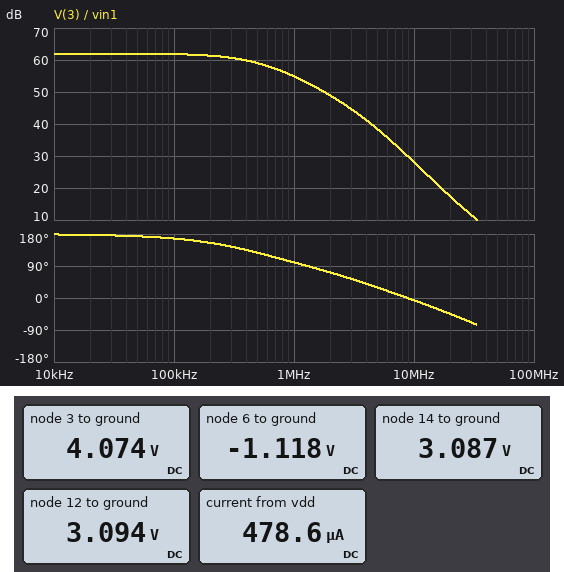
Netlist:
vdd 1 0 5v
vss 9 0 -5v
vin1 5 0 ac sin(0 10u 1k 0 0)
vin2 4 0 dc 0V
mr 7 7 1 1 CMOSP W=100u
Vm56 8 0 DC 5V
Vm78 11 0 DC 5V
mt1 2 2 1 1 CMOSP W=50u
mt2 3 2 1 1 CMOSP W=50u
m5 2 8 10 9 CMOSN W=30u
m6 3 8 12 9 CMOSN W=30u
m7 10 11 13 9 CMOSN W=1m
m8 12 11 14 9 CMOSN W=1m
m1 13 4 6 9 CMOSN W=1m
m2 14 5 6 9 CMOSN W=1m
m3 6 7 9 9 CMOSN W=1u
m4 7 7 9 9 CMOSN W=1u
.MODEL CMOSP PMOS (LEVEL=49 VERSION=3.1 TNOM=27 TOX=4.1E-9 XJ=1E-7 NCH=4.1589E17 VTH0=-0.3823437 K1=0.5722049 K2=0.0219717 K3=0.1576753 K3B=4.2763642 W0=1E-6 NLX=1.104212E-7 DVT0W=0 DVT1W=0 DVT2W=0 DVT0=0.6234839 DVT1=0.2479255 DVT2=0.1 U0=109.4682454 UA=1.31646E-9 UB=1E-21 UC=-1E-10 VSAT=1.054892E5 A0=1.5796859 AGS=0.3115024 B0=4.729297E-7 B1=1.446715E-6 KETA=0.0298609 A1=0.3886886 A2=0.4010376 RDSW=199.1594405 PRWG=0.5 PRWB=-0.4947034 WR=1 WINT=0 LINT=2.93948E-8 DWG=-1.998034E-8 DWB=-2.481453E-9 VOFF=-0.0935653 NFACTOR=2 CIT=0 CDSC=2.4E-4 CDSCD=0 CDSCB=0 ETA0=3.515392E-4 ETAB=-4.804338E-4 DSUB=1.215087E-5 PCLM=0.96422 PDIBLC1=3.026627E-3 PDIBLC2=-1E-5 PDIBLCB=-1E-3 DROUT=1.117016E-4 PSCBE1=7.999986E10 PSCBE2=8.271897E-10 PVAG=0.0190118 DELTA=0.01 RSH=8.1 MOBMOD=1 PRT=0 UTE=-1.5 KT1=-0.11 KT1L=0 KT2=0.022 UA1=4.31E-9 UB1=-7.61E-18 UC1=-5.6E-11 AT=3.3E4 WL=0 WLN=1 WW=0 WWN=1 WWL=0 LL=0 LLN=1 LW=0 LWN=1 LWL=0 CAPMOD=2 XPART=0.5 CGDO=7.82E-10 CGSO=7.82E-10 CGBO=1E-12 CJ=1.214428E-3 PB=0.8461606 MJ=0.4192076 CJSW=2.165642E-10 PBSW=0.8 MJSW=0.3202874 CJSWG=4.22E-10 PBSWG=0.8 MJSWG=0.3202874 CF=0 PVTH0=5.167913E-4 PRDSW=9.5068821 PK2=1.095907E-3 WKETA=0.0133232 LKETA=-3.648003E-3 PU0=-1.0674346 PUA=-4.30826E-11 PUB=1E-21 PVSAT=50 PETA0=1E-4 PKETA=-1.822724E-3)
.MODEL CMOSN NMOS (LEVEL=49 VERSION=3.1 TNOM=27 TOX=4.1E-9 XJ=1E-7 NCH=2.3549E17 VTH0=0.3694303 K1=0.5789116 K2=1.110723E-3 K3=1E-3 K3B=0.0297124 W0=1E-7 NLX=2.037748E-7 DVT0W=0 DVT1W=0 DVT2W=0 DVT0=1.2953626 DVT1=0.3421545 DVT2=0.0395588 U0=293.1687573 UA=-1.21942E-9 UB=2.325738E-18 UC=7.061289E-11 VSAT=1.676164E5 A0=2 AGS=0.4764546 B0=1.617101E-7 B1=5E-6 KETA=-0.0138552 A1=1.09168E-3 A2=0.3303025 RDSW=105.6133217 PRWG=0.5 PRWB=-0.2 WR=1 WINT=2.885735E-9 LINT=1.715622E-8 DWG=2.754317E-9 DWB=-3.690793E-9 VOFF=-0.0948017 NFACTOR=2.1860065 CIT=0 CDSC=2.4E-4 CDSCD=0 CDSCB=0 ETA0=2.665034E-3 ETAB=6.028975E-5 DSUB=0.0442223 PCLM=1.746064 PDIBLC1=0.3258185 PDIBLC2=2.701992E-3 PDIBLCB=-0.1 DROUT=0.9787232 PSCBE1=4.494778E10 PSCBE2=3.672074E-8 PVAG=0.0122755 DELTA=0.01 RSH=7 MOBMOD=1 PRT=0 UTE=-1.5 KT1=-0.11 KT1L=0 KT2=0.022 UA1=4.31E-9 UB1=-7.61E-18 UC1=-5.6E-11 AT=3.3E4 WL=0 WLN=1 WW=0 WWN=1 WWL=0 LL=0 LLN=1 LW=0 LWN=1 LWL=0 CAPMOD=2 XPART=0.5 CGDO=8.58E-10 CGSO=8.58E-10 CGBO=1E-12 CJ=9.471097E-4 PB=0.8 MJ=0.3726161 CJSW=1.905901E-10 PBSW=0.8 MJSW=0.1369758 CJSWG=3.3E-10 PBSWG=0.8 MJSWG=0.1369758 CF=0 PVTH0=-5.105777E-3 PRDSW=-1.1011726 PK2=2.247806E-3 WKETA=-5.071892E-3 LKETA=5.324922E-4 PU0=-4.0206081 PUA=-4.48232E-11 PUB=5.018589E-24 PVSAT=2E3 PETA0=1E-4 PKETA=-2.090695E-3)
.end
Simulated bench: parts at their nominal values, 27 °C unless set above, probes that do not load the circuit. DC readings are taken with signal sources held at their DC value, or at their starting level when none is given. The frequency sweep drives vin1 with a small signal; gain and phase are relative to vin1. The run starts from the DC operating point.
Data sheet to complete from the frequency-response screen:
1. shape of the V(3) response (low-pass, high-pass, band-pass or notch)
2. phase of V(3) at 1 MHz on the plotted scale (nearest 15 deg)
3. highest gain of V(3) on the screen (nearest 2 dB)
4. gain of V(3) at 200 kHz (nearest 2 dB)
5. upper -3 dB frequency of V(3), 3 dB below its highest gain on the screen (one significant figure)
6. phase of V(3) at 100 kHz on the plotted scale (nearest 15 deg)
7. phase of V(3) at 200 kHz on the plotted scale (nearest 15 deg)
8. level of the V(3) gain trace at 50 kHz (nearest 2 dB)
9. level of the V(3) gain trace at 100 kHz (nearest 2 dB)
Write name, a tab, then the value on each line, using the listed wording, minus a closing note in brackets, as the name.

shape of the V(3) response	low-pass
phase of V(3) at 1 MHz on the plotted scale	105 deg
highest gain of V(3) on the screen	62 dB
gain of V(3) at 200 kHz	62 dB
upper -3 dB frequency of V(3), 3 dB below its highest gain on the screen	500 kHz
phase of V(3) at 100 kHz on the plotted scale	165 deg
phase of V(3) at 200 kHz on the plotted scale	150 deg
level of the V(3) gain trace at 50 kHz	62 dB
level of the V(3) gain trace at 100 kHz	62 dB
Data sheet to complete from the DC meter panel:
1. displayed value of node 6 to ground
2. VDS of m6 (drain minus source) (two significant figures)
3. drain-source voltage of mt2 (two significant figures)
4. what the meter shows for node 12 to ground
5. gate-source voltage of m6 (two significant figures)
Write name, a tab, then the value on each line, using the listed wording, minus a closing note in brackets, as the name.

displayed value of node 6 to ground	-1.118 V
VDS of m6 (drain minus source)	980 mV
drain-source voltage of mt2	-930 mV
what the meter shows for node 12 to ground	3.094 V
gate-source voltage of m6	1.9 V
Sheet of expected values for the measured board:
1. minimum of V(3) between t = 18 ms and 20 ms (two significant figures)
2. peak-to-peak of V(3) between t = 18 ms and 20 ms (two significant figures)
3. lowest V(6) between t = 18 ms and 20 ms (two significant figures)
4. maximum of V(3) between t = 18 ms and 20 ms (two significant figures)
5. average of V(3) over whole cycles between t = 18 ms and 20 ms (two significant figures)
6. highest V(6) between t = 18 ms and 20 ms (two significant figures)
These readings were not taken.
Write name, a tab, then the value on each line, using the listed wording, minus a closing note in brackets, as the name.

minimum of V(3) between t = 18 ms and 20 ms	4.1 V
peak-to-peak of V(3) between t = 18 ms and 20 ms	25 mV
lowest V(6) between t = 18 ms and 20 ms	-1.1 V
maximum of V(3) between t = 18 ms and 20 ms	4.1 V
average of V(3) over whole cycles between t = 18 ms and 20 ms	4.1 V
highest V(6) between t = 18 ms and 20 ms	-1.1 V
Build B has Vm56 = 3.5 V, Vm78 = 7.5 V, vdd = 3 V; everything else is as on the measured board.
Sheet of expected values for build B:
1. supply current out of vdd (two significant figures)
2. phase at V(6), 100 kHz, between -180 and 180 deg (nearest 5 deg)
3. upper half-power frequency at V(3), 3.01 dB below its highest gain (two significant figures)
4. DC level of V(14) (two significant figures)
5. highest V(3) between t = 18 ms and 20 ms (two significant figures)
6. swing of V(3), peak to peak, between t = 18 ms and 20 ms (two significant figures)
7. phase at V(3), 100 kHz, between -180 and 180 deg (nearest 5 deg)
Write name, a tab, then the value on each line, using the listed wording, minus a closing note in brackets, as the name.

supply current out of vdd	510 µA
phase at V(6), 100 kHz, between -180 and 180 deg	5 deg
upper half-power frequency at V(3), 3.01 dB below its highest gain	35 kHz
DC level of V(14)	1.7 V
highest V(3) between t = 18 ms and 20 ms	2.0 V
swing of V(3), peak to peak, between t = 18 ms and 20 ms	18 mV
phase at V(3), 100 kHz, between -180 and 180 deg	110 deg
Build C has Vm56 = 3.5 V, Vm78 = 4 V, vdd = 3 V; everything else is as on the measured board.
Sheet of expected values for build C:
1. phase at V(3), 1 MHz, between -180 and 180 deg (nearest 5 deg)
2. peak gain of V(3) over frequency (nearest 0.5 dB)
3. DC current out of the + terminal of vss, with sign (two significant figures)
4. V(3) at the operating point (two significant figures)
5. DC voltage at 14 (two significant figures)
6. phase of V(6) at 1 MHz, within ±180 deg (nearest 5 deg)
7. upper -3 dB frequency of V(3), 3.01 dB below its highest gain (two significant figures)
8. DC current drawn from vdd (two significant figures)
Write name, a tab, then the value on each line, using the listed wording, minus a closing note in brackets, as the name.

phase at V(3), 1 MHz, between -180 and 180 deg	85 deg
peak gain of V(3) over frequency	59.0 dB
DC current out of the + terminal of vss, with sign	-510 µA
V(3) at the operating point	2.0 V
DC voltage at 14	1.7 V
phase of V(6) at 1 MHz, within ±180 deg	0 deg
upper -3 dB frequency of V(3), 3.01 dB below its highest gain	35 kHz
DC current drawn from vdd	510 µA
